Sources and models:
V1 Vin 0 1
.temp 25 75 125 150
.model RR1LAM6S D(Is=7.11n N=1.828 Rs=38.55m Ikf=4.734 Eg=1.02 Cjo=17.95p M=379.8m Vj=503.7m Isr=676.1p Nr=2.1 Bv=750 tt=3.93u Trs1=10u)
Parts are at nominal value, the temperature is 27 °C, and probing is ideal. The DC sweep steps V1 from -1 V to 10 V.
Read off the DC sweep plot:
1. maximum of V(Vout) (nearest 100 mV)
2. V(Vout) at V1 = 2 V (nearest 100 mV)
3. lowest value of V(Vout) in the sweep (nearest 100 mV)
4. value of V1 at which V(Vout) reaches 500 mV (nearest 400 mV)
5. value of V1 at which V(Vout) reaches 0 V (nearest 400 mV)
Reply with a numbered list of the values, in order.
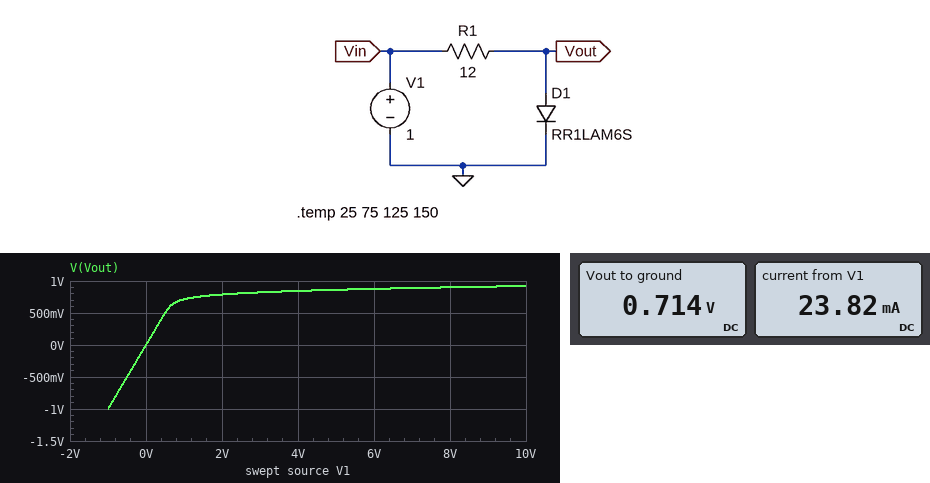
1. 900 mV
2. 800 mV
3. -1.0 V
4. 400 mV
5. 0 V
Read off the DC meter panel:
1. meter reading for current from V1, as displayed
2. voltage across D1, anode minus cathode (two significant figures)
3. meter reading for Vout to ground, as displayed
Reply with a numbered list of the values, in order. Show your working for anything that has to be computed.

1. 23.82 mA
2. 714 mV = 710 mV
3. 0.714 V
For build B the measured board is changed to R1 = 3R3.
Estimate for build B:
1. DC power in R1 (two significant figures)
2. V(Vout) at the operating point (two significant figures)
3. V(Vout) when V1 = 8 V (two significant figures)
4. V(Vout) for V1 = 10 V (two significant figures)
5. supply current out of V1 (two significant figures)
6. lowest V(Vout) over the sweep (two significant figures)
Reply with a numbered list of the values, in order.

1. 16 mW
2. 770 mV
3. 1.0 V
4. 1.1 V
5. 70 mA
6. -1.0 V
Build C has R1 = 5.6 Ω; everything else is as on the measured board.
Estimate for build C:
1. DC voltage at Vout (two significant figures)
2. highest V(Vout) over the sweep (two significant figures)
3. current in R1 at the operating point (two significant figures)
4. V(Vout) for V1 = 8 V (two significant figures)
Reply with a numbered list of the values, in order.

1. 750 mV
2. 1.0 V
3. 45 mA
4. 970 mV
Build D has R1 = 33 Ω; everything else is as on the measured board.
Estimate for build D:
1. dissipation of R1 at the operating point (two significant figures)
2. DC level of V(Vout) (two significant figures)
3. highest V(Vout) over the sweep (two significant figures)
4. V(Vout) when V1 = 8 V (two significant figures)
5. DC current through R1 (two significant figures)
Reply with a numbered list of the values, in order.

1. 3.3 mW
2. 670 mV
3. 850 mV
4. 830 mV
5. 10 mA
